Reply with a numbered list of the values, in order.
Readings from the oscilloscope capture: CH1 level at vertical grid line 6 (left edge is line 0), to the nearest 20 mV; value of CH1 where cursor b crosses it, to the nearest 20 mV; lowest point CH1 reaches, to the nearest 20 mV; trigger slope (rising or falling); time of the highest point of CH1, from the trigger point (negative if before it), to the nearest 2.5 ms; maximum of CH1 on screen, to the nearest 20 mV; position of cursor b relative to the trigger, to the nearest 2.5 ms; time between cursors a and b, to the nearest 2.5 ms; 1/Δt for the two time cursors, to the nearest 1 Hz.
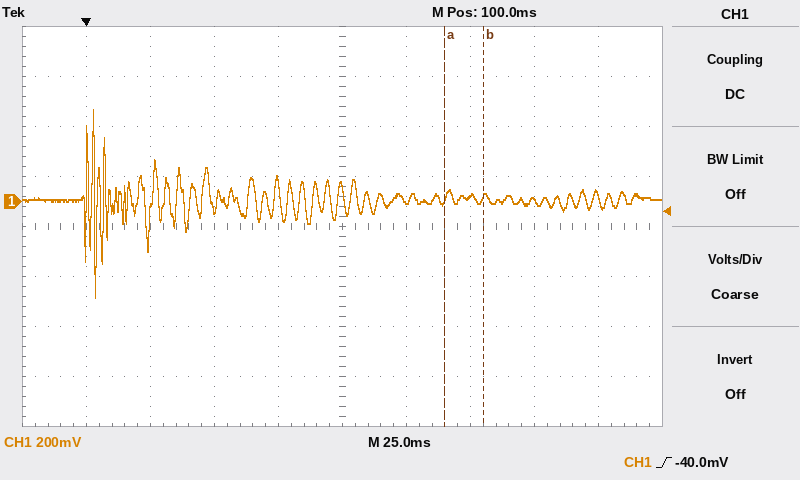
1. 0 mV
2. 20 mV
3. -380 mV
4. rising
5. +2.5 ms
6. 360 mV
7. +155.0 ms
8. 15.0 ms
9. 67 Hz
